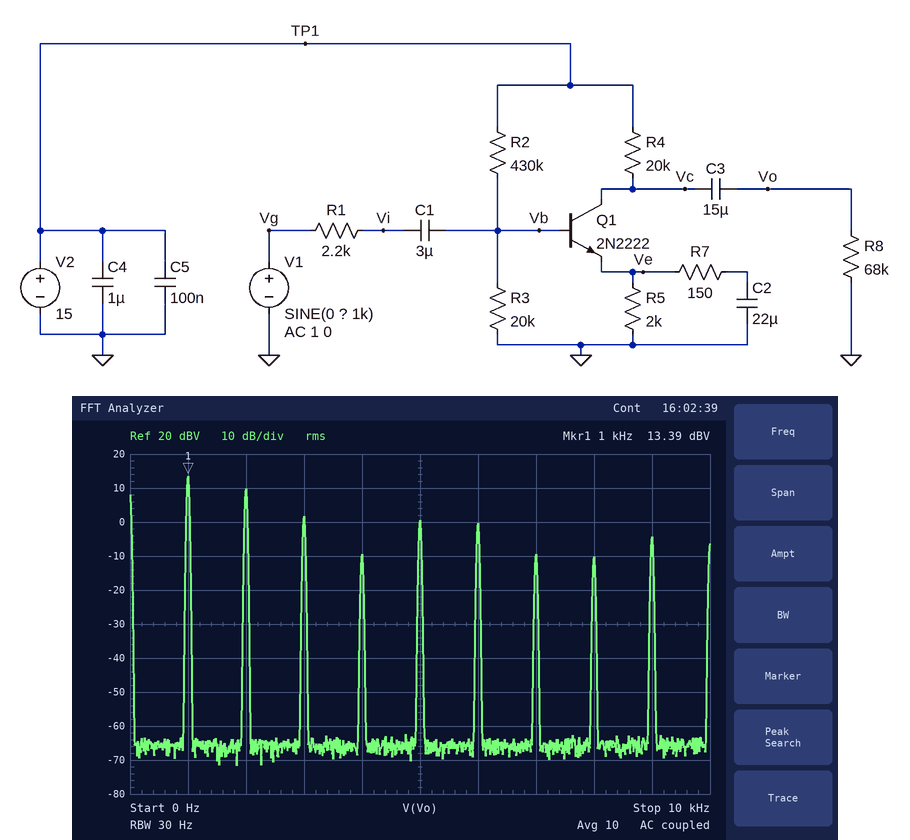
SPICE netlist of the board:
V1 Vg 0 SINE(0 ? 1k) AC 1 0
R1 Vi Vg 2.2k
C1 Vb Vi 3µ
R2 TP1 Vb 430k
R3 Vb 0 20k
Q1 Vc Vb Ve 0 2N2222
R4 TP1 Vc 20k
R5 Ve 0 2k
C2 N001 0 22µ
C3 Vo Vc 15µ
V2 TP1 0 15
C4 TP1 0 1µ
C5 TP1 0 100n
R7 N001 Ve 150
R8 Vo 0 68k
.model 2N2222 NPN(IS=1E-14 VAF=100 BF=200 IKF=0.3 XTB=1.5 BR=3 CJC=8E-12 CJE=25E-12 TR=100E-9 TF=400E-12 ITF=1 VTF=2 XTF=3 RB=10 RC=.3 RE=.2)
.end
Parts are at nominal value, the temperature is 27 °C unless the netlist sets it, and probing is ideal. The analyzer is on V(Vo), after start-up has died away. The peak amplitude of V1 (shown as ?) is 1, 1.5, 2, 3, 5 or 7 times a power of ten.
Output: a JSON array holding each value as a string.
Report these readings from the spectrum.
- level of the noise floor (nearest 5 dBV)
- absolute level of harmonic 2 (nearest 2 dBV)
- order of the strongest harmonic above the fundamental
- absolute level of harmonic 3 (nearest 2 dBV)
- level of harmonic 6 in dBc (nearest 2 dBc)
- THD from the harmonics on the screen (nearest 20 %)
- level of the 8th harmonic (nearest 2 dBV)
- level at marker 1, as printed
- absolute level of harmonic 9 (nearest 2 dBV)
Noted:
["-65 dBV", "10 dBV", "2", "2 dBV", "-14 dBc", "80 %", "-10 dBV", "13.39 dBV", "-4 dBV"]
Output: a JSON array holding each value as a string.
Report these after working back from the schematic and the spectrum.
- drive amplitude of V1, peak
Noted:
["2 V"]
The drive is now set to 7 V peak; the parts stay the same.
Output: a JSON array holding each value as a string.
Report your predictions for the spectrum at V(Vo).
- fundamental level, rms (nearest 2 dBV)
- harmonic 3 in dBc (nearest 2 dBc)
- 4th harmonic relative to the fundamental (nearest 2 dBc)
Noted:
["14 dBV", "-14 dBc", "-18 dBc"]
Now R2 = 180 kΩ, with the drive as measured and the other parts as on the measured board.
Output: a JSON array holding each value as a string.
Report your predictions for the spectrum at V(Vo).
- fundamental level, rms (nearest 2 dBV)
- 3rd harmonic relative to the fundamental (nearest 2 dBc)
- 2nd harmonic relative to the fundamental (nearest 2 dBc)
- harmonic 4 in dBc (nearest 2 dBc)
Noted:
["14 dBV", "-30 dBc", "-6 dBc", "-12 dBc"]
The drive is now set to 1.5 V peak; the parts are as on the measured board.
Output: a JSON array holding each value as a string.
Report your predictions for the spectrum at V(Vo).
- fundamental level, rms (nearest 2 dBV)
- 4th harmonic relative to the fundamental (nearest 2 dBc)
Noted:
["14 dBV", "-28 dBc"]
